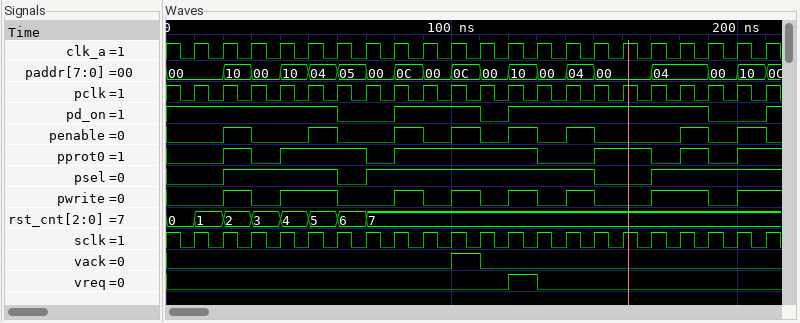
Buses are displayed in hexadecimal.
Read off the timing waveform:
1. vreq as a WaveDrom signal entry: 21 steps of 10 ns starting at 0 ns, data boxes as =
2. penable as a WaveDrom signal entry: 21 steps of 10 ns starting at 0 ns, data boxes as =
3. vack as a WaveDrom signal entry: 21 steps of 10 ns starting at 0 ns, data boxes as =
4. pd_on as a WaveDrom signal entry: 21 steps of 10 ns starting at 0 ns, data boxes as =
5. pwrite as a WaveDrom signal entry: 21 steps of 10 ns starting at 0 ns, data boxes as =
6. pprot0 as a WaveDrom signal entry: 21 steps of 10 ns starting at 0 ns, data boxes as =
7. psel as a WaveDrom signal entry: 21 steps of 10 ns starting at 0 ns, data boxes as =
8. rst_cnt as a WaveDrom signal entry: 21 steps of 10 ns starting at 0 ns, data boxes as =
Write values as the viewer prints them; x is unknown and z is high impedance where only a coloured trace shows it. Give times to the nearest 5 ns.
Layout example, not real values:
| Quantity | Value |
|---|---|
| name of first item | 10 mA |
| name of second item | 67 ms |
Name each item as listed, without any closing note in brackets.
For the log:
| Quantity | Value |
|---|---|
| vreq as a WaveDrom signal entry: 21 steps of 10 ns starting at 0 ns, data boxes as = | {name: 'vreq', wave: '0...........10.......'} |
| penable as a WaveDrom signal entry: 21 steps of 10 ns starting at 0 ns, data boxes as = | {name: 'penable', wave: '0.10.10.10101010..101'} |
| vack as a WaveDrom signal entry: 21 steps of 10 ns starting at 0 ns, data boxes as = | {name: 'vack', wave: '0.........10.........'} |
| pd_on as a WaveDrom signal entry: 21 steps of 10 ns starting at 0 ns, data boxes as = | {name: 'pd_on', wave: '1.....0.1..01......0.'} |
| pwrite as a WaveDrom signal entry: 21 steps of 10 ns starting at 0 ns, data boxes as = | {name: 'pwrite', wave: '0.101.0.10101010.1.01'} |
| pprot0 as a WaveDrom signal entry: 21 steps of 10 ns starting at 0 ns, data boxes as = | {name: 'pprot0', wave: '0.101..01....0.1.0101'} |
| psel as a WaveDrom signal entry: 21 steps of 10 ns starting at 0 ns, data boxes as = | {name: 'psel', wave: '0.1...01.......0.1...'} |
| rst_cnt as a WaveDrom signal entry: 21 steps of 10 ns starting at 0 ns, data boxes as = | {name: 'rst_cnt', wave: '========.............', data: '0 1 2 3 4 5 6 7'} |
